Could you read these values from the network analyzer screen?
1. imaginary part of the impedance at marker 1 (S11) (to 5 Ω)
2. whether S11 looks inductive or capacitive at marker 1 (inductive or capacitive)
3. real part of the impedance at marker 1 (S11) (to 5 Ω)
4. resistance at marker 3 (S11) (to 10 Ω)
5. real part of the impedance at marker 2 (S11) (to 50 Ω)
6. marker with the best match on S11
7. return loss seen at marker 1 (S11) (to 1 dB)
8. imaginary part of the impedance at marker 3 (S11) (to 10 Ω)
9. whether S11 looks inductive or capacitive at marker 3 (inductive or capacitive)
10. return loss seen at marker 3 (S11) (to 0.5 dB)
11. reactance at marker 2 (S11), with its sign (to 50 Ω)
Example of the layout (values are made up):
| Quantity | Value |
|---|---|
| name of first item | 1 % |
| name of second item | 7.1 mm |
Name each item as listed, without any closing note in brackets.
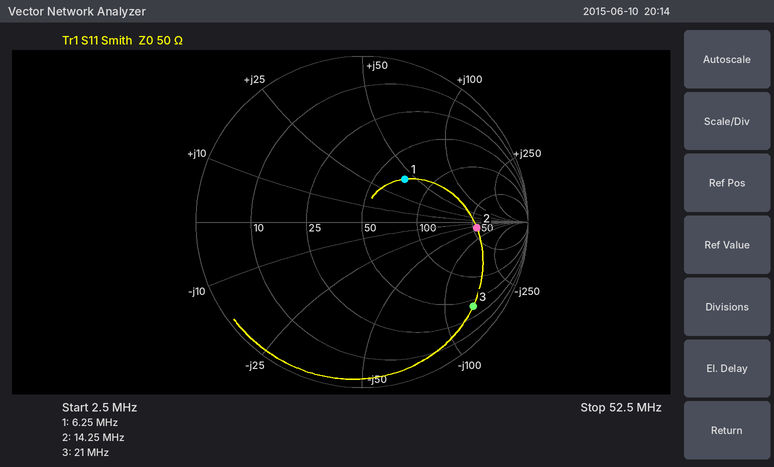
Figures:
| Quantity | Value |
|---|---|
| imaginary part of the impedance at marker 1 (S11) | +40 Ω |
| whether S11 looks inductive or capacitive at marker 1 | inductive |
| real part of the impedance at marker 1 (S11) | 70 Ω |
| resistance at marker 3 (S11) | 40 Ω |
| real part of the impedance at marker 2 (S11) | 250 Ω |
| marker with the best match on S11 | marker 1 |
| return loss seen at marker 1 (S11) | 9 dB |
| imaginary part of the impedance at marker 3 (S11) | -140 Ω |
| whether S11 looks inductive or capacitive at marker 3 | capacitive |
| return loss seen at marker 3 (S11) | 1.5 dB |
| reactance at marker 2 (S11), with its sign | -50 Ω |
